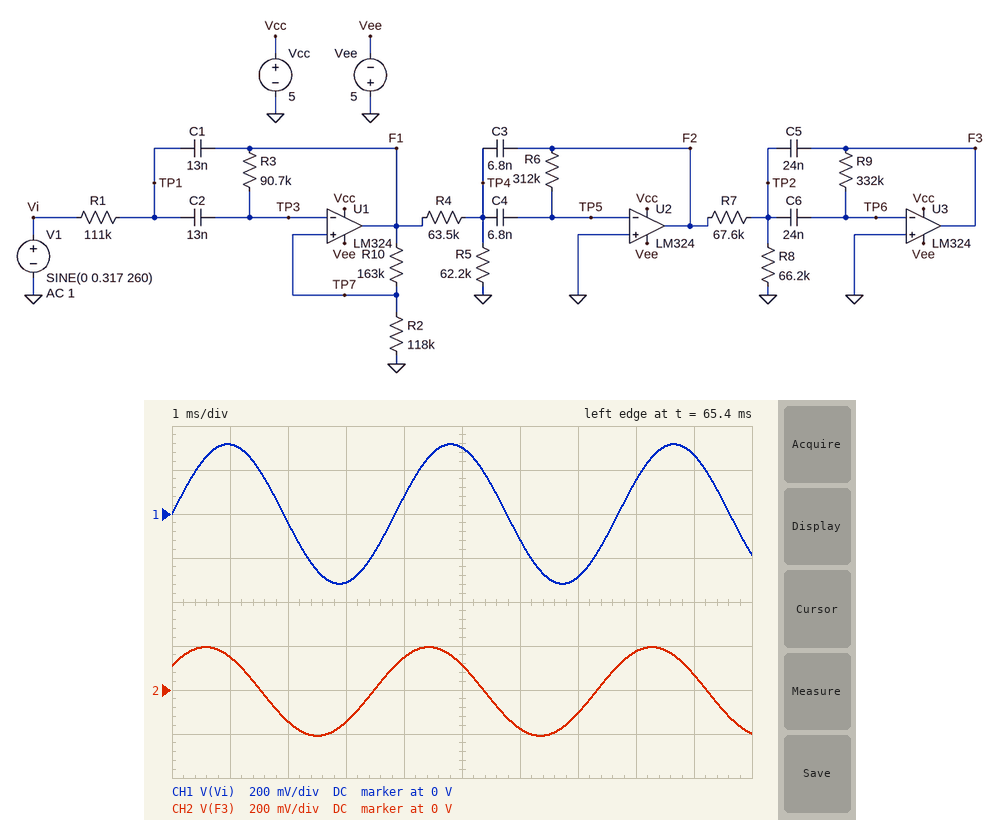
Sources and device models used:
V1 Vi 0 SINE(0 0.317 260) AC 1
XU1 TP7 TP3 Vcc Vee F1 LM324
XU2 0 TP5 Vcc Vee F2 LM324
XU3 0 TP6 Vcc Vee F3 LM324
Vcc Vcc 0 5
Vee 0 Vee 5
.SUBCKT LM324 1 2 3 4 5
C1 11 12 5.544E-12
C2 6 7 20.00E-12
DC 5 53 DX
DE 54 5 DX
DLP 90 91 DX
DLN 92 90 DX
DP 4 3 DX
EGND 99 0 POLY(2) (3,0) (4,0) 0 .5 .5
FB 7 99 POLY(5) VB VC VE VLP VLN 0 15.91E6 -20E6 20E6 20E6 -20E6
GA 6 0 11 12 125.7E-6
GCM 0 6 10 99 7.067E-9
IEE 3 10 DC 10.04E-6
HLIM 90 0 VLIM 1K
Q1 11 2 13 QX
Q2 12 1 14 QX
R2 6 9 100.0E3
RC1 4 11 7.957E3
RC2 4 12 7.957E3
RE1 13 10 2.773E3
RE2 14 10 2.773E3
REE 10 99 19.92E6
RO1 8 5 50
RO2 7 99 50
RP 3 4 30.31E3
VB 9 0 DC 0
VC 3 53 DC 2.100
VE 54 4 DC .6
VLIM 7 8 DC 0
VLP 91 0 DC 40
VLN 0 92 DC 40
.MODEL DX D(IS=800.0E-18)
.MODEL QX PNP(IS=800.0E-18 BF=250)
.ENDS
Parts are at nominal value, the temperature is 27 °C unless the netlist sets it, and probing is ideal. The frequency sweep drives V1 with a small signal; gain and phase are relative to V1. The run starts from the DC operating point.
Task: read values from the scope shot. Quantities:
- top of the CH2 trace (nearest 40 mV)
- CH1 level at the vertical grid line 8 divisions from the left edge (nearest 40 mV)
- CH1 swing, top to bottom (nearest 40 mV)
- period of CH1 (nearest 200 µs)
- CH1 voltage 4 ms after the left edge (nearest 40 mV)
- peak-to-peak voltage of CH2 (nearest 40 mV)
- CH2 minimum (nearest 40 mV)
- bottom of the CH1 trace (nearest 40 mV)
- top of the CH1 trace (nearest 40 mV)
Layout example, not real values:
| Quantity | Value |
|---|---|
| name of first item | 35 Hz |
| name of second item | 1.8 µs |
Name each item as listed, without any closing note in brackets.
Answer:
| Quantity | Value |
|---|---|
| top of the CH2 trace | 200 mV |
| CH1 level at the vertical grid line 8 divisions from the left edge | 160 mV |
| CH1 swing, top to bottom | 640 mV |
| period of CH1 | 3.8 ms |
| CH1 voltage 4 ms after the left edge | 80 mV |
| peak-to-peak voltage of CH2 | 400 mV |
| CH2 minimum | -200 mV |
| bottom of the CH1 trace | -320 mV |
| top of the CH1 trace | 320 mV |
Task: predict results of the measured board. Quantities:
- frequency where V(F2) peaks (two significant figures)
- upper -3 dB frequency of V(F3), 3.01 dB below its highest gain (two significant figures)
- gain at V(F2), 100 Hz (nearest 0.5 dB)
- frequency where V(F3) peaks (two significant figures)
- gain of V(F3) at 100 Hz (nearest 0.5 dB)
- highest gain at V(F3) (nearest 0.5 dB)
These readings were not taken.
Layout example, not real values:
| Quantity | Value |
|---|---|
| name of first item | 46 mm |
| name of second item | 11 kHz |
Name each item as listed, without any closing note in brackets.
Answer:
| Quantity | Value |
|---|---|
| frequency where V(F2) peaks | 220 Hz |
| upper -3 dB frequency of V(F3), 3.01 dB below its highest gain | 250 Hz |
| gain at V(F2), 100 Hz | -2.5 dB |
| frequency where V(F3) peaks | 140 Hz |
| gain of V(F3) at 100 Hz | 0 dB |
| highest gain at V(F3) | 0 dB |
